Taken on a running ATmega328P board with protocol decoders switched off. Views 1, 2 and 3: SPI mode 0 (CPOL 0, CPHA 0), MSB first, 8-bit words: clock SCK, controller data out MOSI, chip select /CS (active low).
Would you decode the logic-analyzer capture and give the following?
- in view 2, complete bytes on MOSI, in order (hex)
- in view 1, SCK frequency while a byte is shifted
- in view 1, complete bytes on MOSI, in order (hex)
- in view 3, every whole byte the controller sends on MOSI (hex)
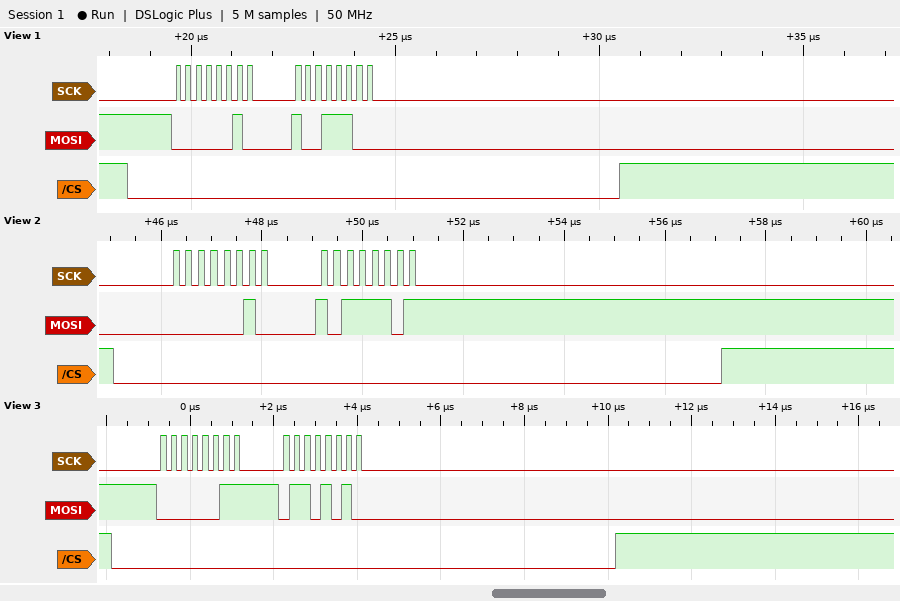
0x02 0xBD
4 MHz
02 9C
03 6A
